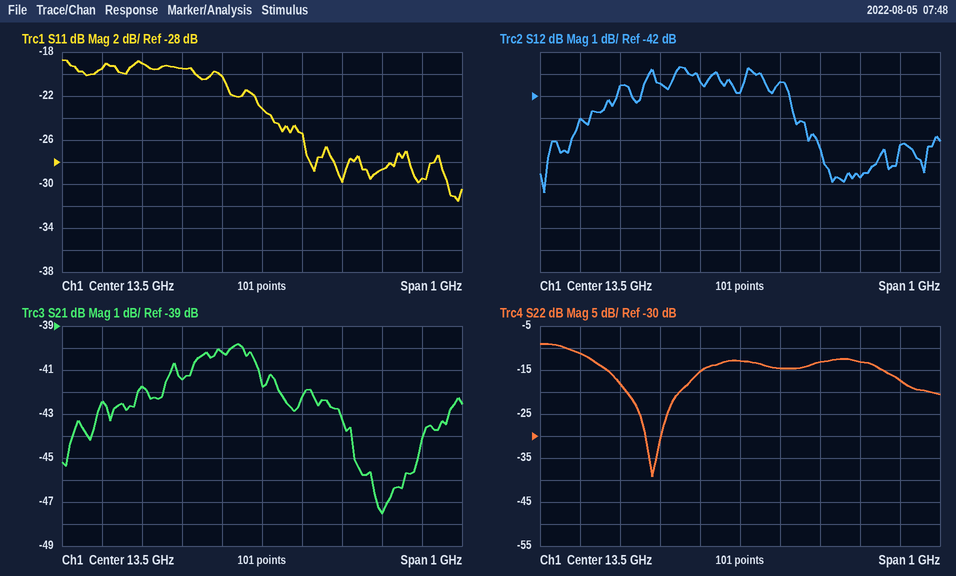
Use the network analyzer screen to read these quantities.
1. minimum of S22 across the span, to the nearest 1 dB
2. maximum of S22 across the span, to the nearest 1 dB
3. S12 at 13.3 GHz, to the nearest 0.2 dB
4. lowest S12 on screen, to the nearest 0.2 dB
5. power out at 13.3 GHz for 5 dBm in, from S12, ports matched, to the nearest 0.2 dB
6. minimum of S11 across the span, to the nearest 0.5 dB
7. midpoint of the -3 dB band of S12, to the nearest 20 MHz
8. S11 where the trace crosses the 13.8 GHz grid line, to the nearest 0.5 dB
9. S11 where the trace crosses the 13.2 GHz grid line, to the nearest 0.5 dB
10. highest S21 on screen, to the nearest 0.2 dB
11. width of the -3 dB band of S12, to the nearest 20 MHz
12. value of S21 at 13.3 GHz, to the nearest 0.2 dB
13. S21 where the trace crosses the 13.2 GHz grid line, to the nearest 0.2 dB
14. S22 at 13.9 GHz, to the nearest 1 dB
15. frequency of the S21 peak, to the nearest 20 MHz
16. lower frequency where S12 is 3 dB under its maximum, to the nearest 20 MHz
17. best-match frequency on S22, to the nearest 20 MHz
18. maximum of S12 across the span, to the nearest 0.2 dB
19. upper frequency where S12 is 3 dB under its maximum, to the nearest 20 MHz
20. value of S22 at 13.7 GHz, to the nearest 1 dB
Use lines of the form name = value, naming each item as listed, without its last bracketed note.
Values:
minimum of S22 across the span, to the nearest 1 dB = -39 dB
maximum of S22 across the span, to the nearest 1 dB = -9 dB
S12 at 13.3 GHz, to the nearest 0.2 dB = -41.4 dB
lowest S12 on screen, to the nearest 0.2 dB = -46.4 dB
power out at 13.3 GHz for 5 dBm in, from S12, ports matched, to the nearest 0.2 dB = -36.4 dBm
minimum of S11 across the span, to the nearest 0.5 dB = -31.5 dB
midpoint of the -3 dB band of S12, to the nearest 20 MHz = 13.38 GHz
S11 where the trace crosses the 13.8 GHz grid line, to the nearest 0.5 dB = -28.5 dB
S11 where the trace crosses the 13.2 GHz grid line, to the nearest 0.5 dB = -19.0 dB
highest S21 on screen, to the nearest 0.2 dB = -39.8 dB
width of the -3 dB band of S12, to the nearest 20 MHz = 580 MHz
value of S21 at 13.3 GHz, to the nearest 0.2 dB = -41.4 dB
S21 where the trace crosses the 13.2 GHz grid line, to the nearest 0.2 dB = -41.8 dB
S22 at 13.9 GHz, to the nearest 1 dB = -17 dB
frequency of the S21 peak, to the nearest 20 MHz = 13.44 GHz
lower frequency where S12 is 3 dB under its maximum, to the nearest 20 MHz = 13.08 GHz
best-match frequency on S22, to the nearest 20 MHz = 13.28 GHz
maximum of S12 across the span, to the nearest 0.2 dB = -40.6 dB
upper frequency where S12 is 3 dB under its maximum, to the nearest 20 MHz = 13.66 GHz
value of S22 at 13.7 GHz, to the nearest 1 dB = -13 dB
